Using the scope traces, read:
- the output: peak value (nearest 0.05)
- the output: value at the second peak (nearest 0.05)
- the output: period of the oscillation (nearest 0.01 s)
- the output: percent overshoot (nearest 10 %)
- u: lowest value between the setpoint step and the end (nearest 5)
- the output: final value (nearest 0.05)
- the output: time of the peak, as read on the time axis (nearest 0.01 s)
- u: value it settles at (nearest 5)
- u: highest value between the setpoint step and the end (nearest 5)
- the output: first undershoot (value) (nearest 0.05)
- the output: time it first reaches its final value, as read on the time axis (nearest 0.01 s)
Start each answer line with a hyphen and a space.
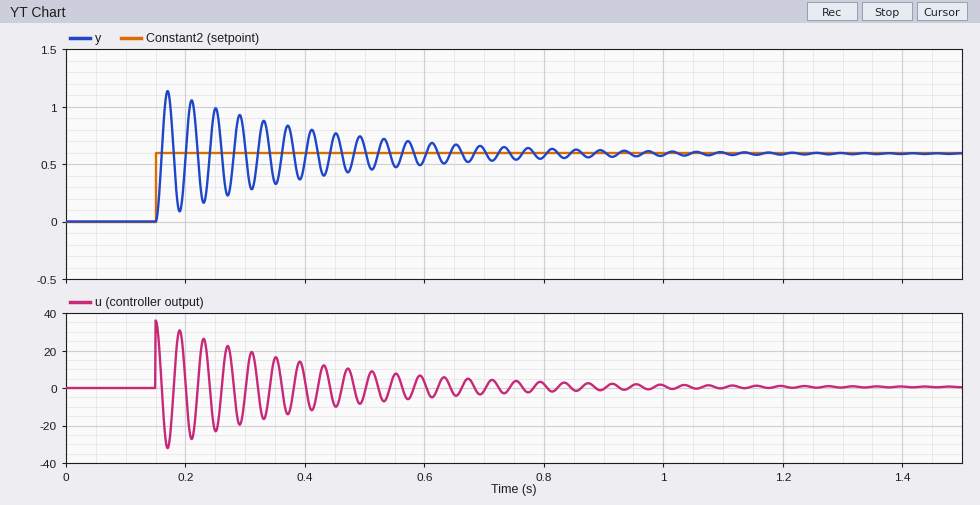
- 1.15
- 1.05
- 0.04 s
- 90 %
- -30
- 0.60
- 0.17 s
- 0
- 35
- 0.10
- 0.16 s
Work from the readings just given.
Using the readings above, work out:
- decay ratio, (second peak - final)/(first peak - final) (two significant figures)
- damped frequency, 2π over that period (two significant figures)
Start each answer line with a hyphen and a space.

- 0.82
- 160 rad/s
